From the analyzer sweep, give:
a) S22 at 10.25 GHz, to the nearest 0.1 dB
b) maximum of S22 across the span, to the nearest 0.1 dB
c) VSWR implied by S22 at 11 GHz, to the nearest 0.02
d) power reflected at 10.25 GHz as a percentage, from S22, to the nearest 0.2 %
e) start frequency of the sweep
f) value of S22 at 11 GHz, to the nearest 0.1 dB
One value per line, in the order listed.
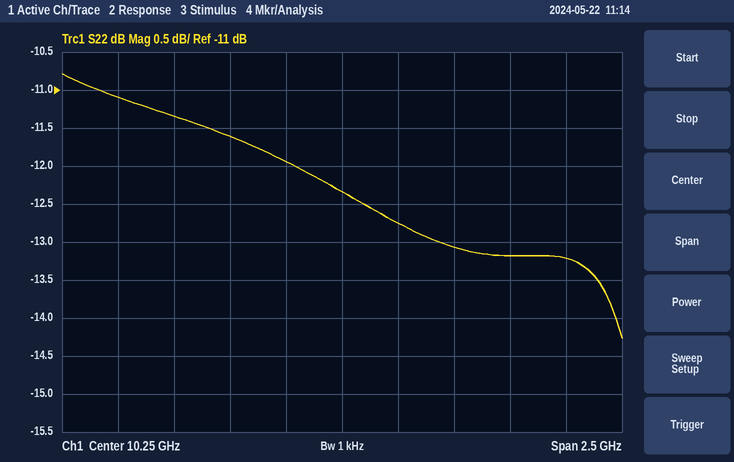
-12.3 dB
-10.8 dB
1.56
5.8 %
9 GHz
-13.2 dB
